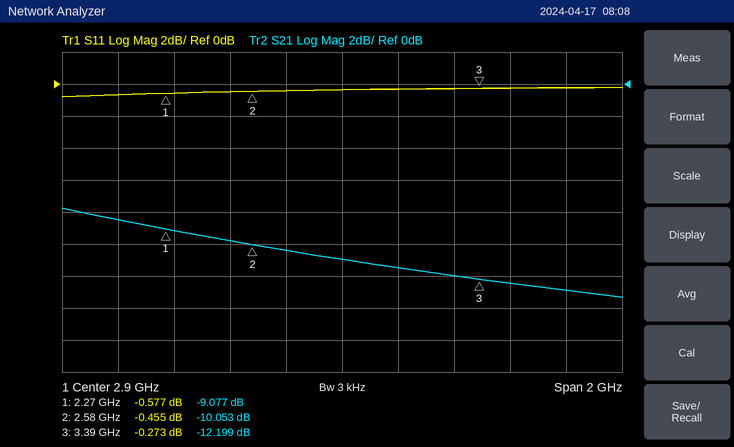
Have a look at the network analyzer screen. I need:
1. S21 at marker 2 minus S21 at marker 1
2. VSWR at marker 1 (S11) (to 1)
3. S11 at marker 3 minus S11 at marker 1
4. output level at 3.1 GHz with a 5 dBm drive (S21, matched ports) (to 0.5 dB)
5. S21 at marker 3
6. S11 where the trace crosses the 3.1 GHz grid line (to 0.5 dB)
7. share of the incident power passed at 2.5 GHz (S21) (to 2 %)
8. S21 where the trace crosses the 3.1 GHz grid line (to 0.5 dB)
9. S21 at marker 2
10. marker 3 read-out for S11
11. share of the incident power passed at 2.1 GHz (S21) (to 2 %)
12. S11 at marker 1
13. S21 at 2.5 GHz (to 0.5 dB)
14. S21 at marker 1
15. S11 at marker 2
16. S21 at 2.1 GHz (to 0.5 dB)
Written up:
-0.976 dB
30
0.304 dB
-6.5 dBm
-12.199 dB
-0.5 dB
10 %
-11.5 dB
-10.053 dB
-0.273 dB
14 %
-0.577 dB
-10.0 dB
-9.077 dB
-0.455 dB
-8.5 dB
